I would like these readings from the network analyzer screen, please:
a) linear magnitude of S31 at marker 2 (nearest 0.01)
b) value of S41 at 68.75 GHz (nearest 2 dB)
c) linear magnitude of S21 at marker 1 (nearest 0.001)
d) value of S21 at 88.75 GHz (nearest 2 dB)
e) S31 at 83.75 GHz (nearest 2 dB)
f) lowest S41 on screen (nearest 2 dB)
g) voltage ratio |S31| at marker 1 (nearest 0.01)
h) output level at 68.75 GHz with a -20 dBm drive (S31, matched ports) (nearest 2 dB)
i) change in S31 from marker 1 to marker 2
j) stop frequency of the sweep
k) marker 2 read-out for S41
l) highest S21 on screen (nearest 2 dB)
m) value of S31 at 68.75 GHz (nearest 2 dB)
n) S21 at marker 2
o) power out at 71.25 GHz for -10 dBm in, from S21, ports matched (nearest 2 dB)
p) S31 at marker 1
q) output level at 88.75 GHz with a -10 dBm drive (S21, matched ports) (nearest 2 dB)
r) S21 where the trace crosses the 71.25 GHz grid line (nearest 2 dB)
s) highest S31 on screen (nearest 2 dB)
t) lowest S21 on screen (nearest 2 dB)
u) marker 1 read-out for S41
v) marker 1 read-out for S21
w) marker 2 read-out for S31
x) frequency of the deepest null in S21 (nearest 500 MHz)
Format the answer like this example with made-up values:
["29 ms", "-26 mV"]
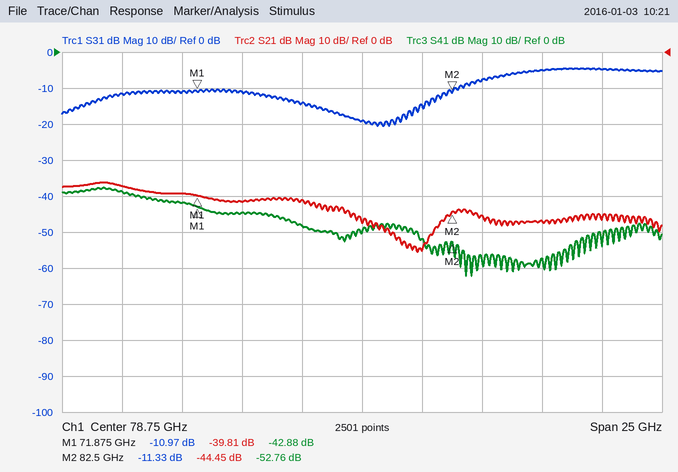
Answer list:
["0.27", "-38 dB", "0.010", "-46 dB", "-8 dB", "-62 dB", "0.28", "-32 dBm", "-0.36 dB", "91.25 GHz", "-52.76 dB", "-36 dB", "-12 dB", "-44.45 dB", "-50 dBm", "-10.97 dB", "-56 dBm", "-40 dB", "-4 dB", "-56 dB", "-42.88 dB", "-39.81 dB", "-11.33 dB", "81.0 GHz"]
